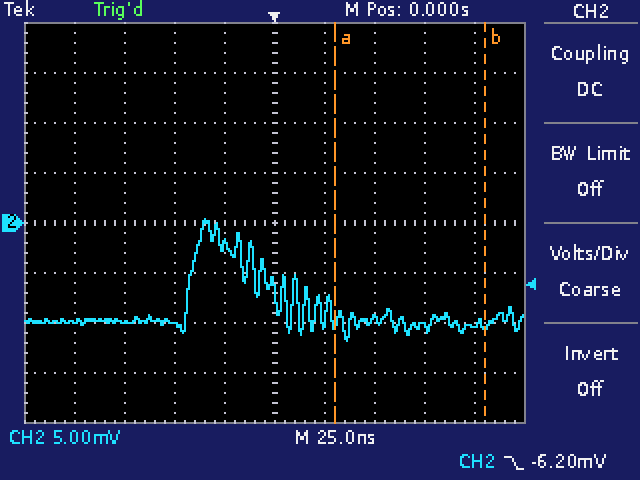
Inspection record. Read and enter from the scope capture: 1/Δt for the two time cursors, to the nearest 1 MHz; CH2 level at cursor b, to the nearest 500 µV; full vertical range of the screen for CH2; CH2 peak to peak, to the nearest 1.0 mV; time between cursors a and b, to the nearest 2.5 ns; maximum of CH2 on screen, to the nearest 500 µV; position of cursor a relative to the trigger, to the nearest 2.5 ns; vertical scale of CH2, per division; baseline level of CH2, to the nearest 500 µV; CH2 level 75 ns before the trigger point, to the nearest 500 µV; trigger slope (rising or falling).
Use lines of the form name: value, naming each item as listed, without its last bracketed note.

1/Δt for the two time cursors, to the nearest 1 MHz: 13 MHz
CH2 level at cursor b, to the nearest 500 µV: -10.0 mV
full vertical range of the screen for CH2: 40 mV
CH2 peak to peak, to the nearest 1.0 mV: 12.0 mV
time between cursors a and b, to the nearest 2.5 ns: 75.0 ns
maximum of CH2 on screen, to the nearest 500 µV: 500 µV
position of cursor a relative to the trigger, to the nearest 2.5 ns: +30.0 ns
vertical scale of CH2, per division: 5 mV
baseline level of CH2, to the nearest 500 µV: -10.0 mV
CH2 level 75 ns before the trigger point, to the nearest 500 µV: -10.0 mV
trigger slope: falling
